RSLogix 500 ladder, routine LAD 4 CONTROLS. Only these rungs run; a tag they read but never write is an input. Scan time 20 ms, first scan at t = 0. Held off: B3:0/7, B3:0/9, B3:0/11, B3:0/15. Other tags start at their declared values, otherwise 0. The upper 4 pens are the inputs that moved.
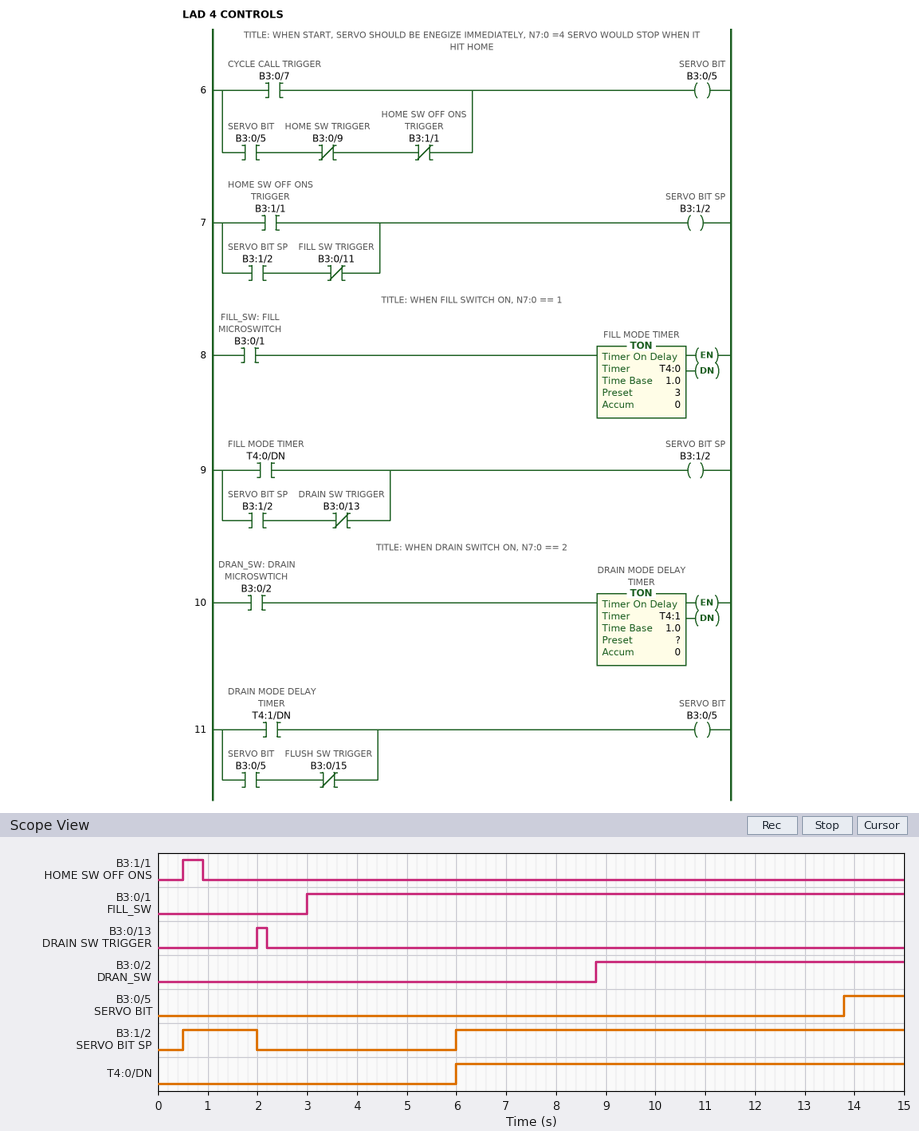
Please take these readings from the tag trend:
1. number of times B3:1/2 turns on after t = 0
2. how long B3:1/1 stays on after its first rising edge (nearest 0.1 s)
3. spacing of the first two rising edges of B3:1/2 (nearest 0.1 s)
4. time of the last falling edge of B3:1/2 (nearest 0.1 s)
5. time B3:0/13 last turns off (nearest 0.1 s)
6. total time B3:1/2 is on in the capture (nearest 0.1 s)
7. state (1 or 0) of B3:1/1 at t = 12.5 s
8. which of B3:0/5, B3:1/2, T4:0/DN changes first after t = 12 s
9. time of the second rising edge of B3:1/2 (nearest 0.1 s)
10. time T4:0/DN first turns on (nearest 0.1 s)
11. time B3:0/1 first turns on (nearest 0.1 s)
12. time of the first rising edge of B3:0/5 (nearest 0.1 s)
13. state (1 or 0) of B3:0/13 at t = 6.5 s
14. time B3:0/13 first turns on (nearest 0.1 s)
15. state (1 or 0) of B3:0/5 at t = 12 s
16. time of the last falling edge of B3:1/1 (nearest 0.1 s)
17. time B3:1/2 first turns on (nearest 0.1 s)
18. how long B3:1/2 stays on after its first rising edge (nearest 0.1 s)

2
0.4 s
5.5 s
2.0 s
2.2 s
10.5 s
0
B3:0/5
6.0 s
6.0 s
3.0 s
13.8 s
0
2.0 s
0
0.9 s
0.5 s
1.5 s
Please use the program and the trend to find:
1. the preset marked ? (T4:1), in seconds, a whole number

5 s
